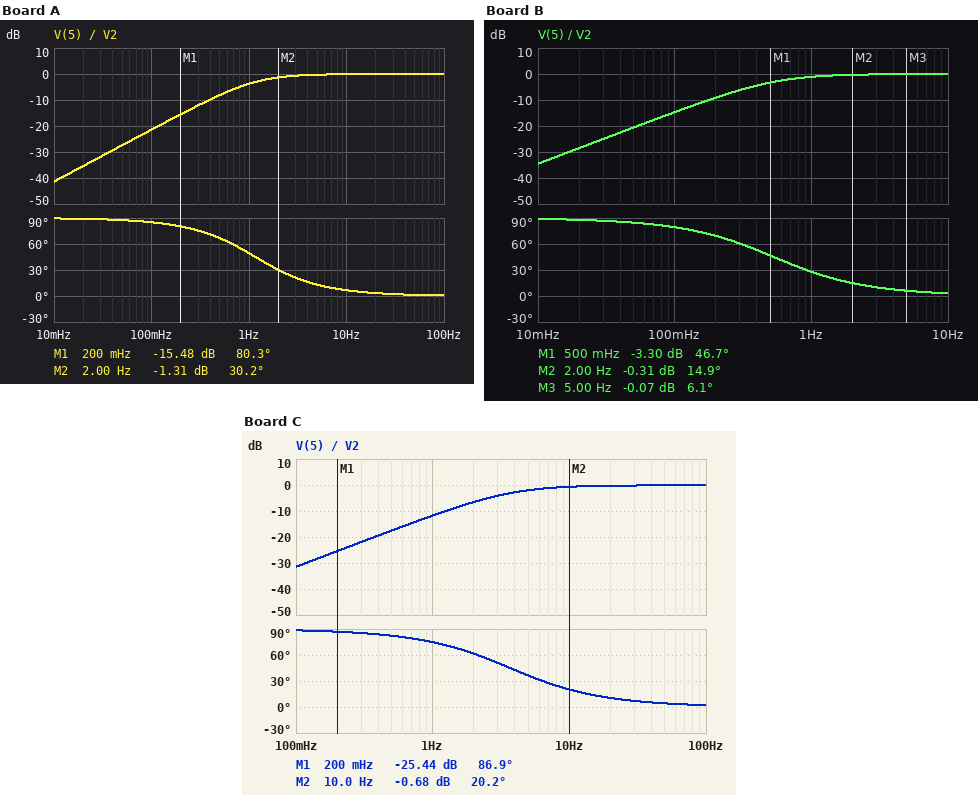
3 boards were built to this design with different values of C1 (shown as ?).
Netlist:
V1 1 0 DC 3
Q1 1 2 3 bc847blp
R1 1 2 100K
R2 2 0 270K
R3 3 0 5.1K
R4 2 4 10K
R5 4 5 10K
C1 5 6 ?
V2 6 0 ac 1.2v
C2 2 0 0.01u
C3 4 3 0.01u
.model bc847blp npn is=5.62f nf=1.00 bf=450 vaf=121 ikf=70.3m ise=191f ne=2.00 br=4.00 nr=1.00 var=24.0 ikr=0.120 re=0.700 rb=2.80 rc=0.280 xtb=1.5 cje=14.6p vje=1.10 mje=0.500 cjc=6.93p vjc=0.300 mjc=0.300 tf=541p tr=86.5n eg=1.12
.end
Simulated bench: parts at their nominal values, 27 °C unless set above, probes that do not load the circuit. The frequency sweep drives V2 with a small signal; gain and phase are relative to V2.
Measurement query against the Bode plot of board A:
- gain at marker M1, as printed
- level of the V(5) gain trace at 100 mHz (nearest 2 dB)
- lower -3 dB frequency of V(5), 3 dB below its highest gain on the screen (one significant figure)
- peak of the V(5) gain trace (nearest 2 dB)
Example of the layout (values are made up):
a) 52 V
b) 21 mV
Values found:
a) -15.48 dB
b) -22 dB
c) 1 Hz
d) 0 dB
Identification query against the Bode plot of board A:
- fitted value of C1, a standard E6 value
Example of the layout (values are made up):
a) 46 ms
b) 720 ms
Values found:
a) 1.5 µF
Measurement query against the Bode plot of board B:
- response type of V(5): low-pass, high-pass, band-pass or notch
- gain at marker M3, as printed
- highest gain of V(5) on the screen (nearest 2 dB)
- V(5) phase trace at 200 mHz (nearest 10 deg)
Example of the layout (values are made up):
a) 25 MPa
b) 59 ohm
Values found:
a) high-pass
b) -0.07 dB
c) 0 dB
d) 70 deg
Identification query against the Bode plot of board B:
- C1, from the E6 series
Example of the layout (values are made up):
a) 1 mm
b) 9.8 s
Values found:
a) 3.3 µF
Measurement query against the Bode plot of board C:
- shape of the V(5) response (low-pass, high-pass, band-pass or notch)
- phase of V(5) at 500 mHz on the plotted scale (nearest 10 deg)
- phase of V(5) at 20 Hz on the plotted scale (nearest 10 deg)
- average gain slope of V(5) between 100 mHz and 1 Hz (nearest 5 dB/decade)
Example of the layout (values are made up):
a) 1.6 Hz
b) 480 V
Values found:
a) high-pass
b) 80 deg
c) 10 deg
d) 20 dB/decade
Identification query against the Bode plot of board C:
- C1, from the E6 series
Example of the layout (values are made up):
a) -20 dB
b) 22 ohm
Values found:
a) 470 nF
